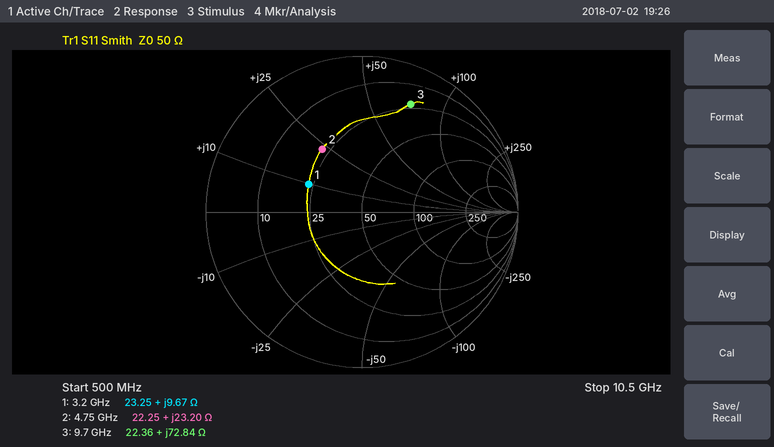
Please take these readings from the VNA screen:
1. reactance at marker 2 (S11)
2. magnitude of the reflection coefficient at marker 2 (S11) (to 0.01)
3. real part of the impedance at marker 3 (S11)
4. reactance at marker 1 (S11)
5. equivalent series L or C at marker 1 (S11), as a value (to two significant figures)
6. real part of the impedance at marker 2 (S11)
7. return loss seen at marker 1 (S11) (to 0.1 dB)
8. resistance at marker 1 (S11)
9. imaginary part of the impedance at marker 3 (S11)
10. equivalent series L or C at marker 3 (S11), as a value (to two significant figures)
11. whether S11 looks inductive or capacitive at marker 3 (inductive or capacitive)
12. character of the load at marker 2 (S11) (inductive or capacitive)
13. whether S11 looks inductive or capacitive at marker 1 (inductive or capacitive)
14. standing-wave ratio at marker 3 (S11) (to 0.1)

+23.20 Ω
0.48
22.36 Ω
+9.67 Ω
480 pH
22.25 Ω
8.3 dB
23.25 Ω
+72.84 Ω
1.2 nH
inductive
inductive
inductive
7.3
